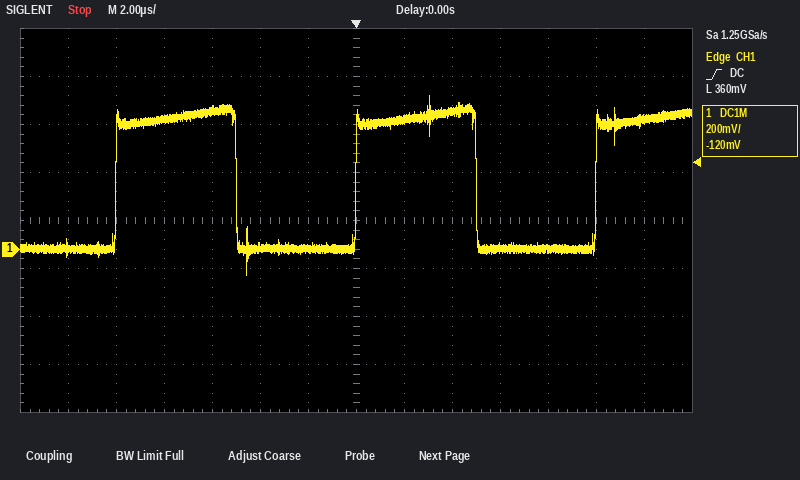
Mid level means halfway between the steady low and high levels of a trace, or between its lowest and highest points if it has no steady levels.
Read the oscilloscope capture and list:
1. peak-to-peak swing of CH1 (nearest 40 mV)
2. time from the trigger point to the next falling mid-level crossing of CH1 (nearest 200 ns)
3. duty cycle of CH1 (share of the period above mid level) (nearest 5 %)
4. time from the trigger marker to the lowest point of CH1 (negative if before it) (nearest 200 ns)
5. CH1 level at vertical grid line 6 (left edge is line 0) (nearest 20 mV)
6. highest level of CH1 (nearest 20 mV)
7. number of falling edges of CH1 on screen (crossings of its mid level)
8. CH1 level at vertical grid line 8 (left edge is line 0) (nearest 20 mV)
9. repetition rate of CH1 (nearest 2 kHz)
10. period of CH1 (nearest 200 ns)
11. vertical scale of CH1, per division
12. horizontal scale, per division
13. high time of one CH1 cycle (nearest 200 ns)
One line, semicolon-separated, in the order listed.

760 mV; 5.0 µs; 50 %; -4.6 µs; 0 mV; 640 mV; 2; 540 mV; 100 kHz; 10.0 µs; 200 mV; 2 µs; 5.0 µs
